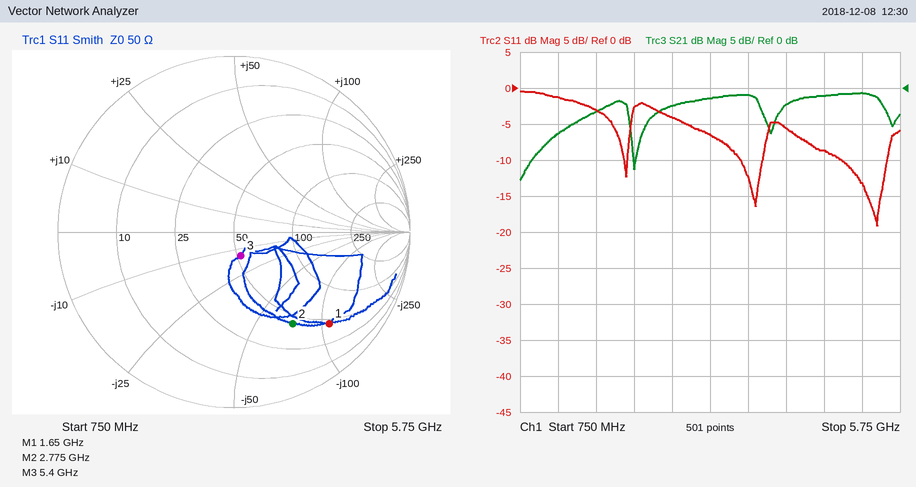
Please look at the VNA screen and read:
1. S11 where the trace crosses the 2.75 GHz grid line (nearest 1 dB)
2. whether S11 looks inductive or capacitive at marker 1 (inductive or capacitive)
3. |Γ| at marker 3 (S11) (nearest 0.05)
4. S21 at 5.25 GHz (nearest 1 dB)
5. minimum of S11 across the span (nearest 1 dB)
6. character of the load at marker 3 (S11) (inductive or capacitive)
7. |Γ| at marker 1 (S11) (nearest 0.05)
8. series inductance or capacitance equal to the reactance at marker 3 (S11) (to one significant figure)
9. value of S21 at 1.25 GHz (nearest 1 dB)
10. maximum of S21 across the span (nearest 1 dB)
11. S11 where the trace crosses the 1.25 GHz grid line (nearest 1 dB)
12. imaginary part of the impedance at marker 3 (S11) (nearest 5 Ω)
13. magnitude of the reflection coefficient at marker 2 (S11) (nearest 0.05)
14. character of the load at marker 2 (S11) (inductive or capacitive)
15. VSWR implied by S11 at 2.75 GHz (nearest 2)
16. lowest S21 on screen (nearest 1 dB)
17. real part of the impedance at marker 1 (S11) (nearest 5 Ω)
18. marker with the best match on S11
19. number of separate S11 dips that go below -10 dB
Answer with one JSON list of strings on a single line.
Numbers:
["-4 dB", "capacitive", "0.15", "-1 dB", "-19 dB", "capacitive", "0.75", "2 pF", "-6 dB", "-1 dB", "-1 dB", "-15 Ω", "0.60", "capacitive", "4", "-13 dB", "45 Ω", "marker 3", "3"]
